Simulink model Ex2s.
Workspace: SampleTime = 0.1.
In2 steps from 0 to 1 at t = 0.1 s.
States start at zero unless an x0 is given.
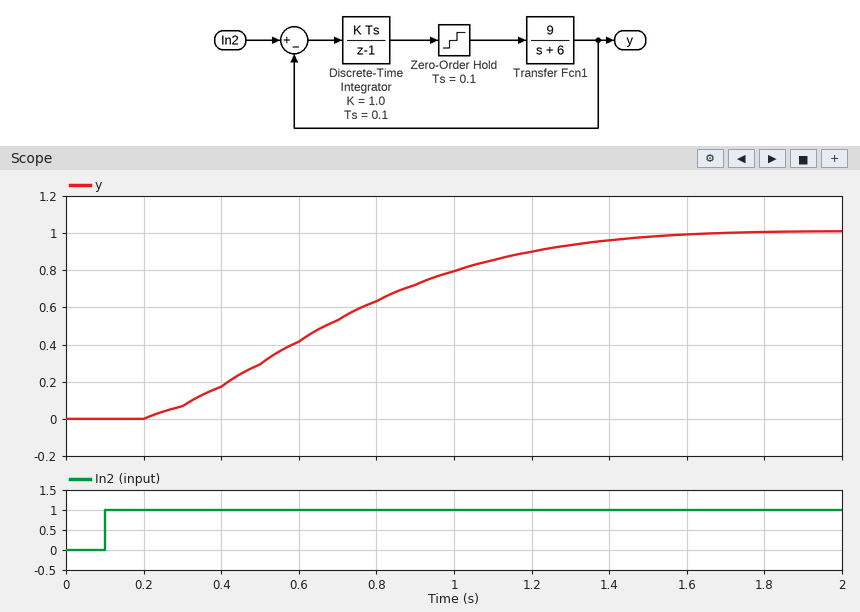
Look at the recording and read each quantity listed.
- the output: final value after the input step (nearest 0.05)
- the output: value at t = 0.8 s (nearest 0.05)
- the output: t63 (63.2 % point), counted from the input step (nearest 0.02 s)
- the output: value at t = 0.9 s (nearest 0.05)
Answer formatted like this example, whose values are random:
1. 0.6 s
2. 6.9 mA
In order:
1. 1.00
2. 0.65
3. 0.70 s
4. 0.70
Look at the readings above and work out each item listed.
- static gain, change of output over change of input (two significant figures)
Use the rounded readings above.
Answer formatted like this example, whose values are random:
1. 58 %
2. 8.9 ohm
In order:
1. 1.0
